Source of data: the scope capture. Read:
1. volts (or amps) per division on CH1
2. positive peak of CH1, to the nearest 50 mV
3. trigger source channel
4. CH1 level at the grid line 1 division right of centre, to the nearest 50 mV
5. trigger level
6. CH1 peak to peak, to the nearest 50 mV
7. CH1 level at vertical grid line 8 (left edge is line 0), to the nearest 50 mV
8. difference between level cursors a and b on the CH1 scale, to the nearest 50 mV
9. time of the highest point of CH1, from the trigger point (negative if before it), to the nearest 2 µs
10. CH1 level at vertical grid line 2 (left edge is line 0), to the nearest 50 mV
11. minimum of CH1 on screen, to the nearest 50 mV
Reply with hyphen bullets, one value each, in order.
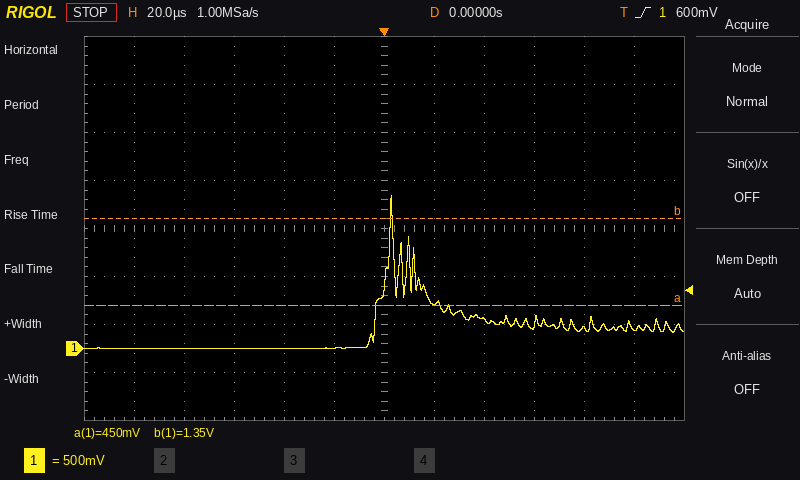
- 500 mV
- 1.60 V
- CH1
- 450 mV
- 600 mV
- 1.60 V
- 300 mV
- 900 mV
- +2 µs
- 0 mV
- 0 mV
